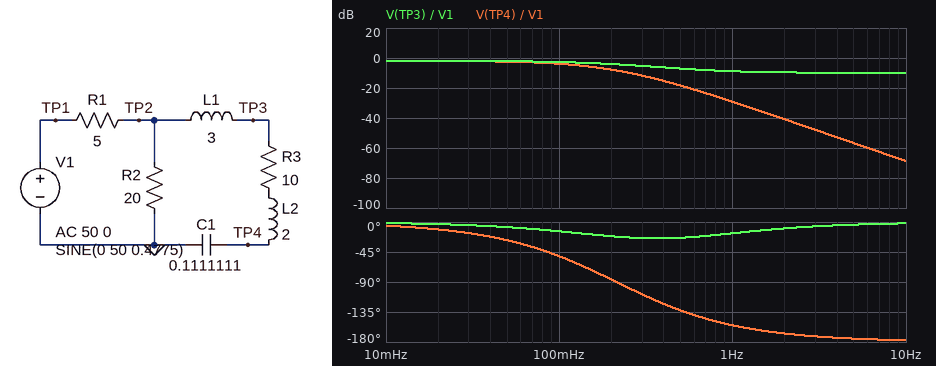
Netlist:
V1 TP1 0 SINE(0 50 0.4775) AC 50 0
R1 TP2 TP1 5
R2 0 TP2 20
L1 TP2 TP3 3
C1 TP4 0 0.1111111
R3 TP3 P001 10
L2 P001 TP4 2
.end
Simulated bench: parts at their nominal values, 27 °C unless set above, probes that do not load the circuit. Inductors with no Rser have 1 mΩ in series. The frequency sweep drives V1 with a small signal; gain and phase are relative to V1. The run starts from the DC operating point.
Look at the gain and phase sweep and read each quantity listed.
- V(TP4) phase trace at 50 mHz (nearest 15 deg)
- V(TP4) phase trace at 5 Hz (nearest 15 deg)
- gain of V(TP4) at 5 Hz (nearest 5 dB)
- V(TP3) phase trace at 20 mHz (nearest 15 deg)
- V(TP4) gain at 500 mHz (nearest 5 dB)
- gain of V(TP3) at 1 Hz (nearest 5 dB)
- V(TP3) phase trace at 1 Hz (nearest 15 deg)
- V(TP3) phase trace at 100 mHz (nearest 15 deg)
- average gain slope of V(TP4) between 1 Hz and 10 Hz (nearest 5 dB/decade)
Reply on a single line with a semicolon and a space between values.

-30 deg; -180 deg; -55 dB; 0 deg; -20 dB; -10 dB; -15 deg; -15 deg; -40 dB/decade
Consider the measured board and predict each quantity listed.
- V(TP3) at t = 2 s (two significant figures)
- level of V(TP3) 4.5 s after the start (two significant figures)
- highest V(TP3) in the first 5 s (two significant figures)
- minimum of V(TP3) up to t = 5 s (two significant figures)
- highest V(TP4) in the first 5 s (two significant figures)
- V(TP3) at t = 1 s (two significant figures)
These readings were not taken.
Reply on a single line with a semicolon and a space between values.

-14 V; 11 V; 26 V; -23 V; 12 V; 14 V
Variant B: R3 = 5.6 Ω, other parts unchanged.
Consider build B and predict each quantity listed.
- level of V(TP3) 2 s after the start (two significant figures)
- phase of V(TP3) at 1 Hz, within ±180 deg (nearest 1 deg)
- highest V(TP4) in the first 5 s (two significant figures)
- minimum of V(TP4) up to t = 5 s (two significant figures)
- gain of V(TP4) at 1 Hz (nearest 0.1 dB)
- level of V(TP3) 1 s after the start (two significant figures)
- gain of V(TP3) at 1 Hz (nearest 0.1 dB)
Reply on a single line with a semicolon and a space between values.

-9.5 V; -9 deg; 15 V; -8.1 V; -28.8 dB; 13 V; -10.0 dB
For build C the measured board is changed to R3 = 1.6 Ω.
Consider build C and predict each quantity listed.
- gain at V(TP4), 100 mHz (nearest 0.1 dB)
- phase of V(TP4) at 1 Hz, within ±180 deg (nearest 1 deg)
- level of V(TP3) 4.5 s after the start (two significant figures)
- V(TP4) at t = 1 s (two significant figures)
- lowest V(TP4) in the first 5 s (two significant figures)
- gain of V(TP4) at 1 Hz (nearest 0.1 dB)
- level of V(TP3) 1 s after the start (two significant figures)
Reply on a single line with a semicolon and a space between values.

-0.8 dB; -169 deg; 7.1 V; 15 V; -10 V; -28.5 dB; 9.8 V
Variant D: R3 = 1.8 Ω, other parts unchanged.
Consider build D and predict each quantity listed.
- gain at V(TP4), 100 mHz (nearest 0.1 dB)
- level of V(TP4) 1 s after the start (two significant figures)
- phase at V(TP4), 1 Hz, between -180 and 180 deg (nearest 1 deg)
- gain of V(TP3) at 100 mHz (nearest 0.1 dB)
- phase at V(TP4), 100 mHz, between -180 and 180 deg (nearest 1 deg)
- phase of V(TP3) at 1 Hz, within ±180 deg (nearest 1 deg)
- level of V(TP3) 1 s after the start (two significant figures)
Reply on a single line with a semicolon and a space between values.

-0.8 dB; 15 V; -169 deg; -1.5 dB; -27 deg; 2 deg; 10 V
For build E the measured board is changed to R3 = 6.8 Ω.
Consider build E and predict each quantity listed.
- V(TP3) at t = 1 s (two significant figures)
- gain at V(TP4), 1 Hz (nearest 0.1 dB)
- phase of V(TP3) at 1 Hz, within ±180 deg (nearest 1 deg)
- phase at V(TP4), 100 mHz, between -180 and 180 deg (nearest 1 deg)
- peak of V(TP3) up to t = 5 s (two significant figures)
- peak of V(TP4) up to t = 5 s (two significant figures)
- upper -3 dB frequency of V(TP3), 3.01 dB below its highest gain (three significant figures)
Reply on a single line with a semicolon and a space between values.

13 V; -28.9 dB; -12 deg; -44 deg; 23 V; 14 V; 226 mHz
